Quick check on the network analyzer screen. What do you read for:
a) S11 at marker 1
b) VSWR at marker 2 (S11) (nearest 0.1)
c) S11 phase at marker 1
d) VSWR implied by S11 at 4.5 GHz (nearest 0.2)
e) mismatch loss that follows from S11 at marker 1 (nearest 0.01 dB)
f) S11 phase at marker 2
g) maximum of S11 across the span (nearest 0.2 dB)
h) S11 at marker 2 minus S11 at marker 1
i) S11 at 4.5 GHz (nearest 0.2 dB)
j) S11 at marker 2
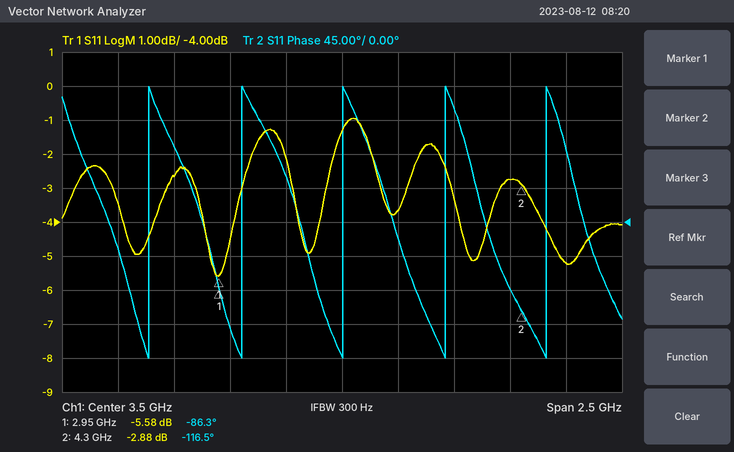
-5.58 dB
6.1
-86.3°
3.4
1.41 dB
-116.5°
-1.0 dB
2.70 dB
-5.2 dB
-2.88 dB
